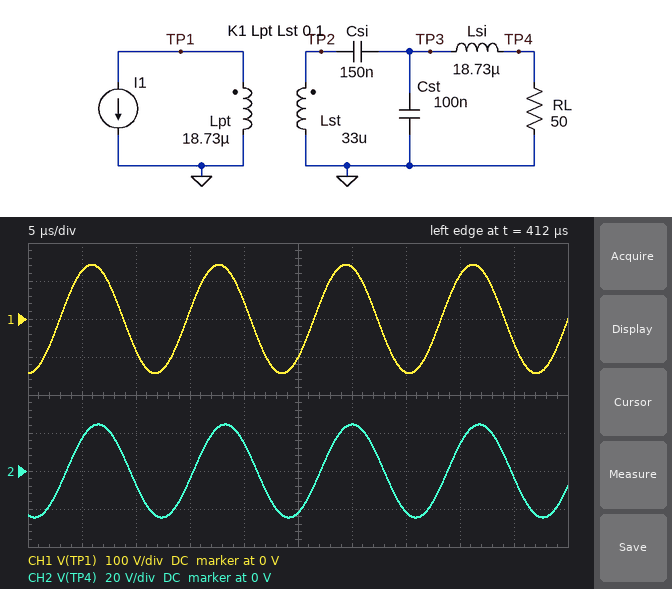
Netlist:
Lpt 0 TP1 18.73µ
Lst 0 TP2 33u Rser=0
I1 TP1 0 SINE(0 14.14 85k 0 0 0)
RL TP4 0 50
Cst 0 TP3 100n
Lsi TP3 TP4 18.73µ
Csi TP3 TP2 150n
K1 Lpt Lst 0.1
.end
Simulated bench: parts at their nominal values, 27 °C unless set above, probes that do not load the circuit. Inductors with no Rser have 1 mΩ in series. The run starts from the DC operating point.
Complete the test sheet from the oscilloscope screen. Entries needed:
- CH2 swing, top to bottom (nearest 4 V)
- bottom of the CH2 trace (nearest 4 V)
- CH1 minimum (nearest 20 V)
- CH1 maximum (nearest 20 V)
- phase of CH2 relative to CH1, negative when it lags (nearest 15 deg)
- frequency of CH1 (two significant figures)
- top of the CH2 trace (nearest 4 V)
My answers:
48 V
-24 V
-140 V
140 V
-15 deg
85 kHz
24 V
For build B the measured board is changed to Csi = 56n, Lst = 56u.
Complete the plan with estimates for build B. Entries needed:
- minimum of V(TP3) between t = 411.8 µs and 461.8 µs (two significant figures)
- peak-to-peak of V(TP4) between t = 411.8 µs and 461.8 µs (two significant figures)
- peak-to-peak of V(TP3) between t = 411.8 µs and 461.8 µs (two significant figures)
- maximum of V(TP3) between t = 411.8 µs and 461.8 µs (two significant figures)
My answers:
-21 V
41 V
42 V
21 V
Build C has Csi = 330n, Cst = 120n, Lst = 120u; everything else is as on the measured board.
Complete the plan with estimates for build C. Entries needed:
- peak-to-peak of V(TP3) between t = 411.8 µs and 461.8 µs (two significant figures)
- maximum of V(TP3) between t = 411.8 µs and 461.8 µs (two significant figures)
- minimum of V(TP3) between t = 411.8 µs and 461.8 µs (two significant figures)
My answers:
26 V
13 V
-13 V
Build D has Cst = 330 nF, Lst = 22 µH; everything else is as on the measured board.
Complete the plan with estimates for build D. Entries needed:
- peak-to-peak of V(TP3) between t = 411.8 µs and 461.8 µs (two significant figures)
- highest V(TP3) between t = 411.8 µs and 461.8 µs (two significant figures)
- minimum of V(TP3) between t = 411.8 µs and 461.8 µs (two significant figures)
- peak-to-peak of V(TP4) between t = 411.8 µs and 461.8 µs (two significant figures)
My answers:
28 V
14 V
-14 V
27 V
